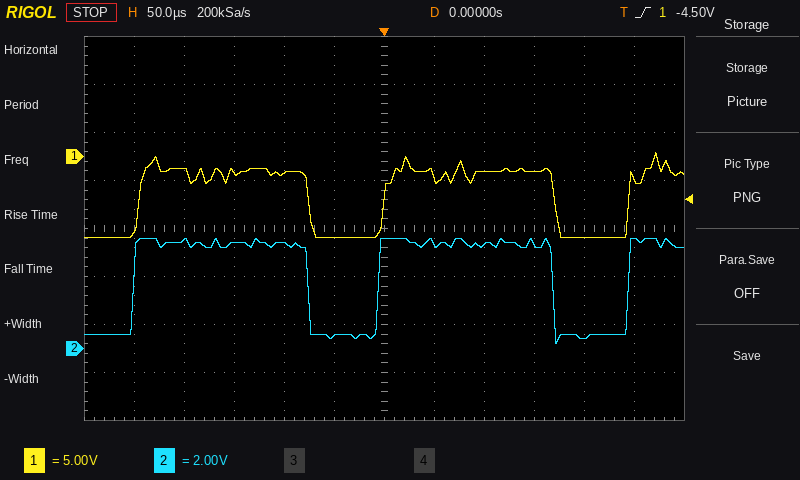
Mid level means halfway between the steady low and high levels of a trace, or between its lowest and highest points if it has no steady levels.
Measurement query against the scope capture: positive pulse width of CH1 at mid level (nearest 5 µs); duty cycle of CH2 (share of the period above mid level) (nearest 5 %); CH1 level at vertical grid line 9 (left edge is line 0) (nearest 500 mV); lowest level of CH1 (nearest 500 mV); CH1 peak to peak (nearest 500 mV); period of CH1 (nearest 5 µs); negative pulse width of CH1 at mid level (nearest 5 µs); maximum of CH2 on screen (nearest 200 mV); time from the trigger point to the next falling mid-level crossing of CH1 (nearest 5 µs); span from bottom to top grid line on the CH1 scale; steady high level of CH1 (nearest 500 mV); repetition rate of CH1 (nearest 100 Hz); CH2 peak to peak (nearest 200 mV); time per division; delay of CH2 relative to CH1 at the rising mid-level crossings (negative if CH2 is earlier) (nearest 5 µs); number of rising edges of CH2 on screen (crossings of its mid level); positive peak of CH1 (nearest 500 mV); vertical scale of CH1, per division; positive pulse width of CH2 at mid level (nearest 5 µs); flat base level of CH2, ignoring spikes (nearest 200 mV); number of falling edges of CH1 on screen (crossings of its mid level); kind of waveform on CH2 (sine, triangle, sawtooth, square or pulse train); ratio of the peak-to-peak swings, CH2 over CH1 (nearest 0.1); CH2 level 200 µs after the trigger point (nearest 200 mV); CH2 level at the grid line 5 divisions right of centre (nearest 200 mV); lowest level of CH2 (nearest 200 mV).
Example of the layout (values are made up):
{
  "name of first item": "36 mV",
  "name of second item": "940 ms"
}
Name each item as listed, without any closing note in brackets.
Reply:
{
  "positive pulse width of CH1 at mid level": "170 µs",
  "duty cycle of CH2 (share of the period above mid level)": "70 %",
  "CH1 level at vertical grid line 9 (left edge is line 0)": "-1.5 V",
  "lowest level of CH1": "-8.5 V",
  "CH1 peak to peak": "9.0 V",
  "period of CH1": "245 µs",
  "negative pulse width of CH1 at mid level": "75 µs",
  "maximum of CH2 on screen": "4.6 V",
  "time from the trigger point to the next falling mid-level crossing of CH1": "170 µs",
  "span from bottom to top grid line on the CH1 scale": "40 V",
  "steady high level of CH1": "-1.5 V",
  "repetition rate of CH1": "4.1 kHz",
  "CH2 peak to peak": "4.4 V",
  "time per division": "50 µs",
  "delay of CH2 relative to CH1 at the rising mid-level crossings (negative if CH2 is earlier)": "-5 µs",
  "number of rising edges of CH2 on screen": "3",
  "positive peak of CH1": "500 mV",
  "vertical scale of CH1, per division": "5 V",
  "positive pulse width of CH2 at mid level": "175 µs",
  "flat base level of CH2, ignoring spikes": "600 mV",
  "number of falling edges of CH1 on screen": "2",
  "kind of waveform on CH2": "pulse train",
  "ratio of the peak-to-peak swings, CH2 over CH1": "0.5",
  "CH2 level 200 µs after the trigger point": "400 mV",
  "CH2 level at the grid line 5 divisions right of centre": "4.6 V",
  "lowest level of CH2": "200 mV"
}
